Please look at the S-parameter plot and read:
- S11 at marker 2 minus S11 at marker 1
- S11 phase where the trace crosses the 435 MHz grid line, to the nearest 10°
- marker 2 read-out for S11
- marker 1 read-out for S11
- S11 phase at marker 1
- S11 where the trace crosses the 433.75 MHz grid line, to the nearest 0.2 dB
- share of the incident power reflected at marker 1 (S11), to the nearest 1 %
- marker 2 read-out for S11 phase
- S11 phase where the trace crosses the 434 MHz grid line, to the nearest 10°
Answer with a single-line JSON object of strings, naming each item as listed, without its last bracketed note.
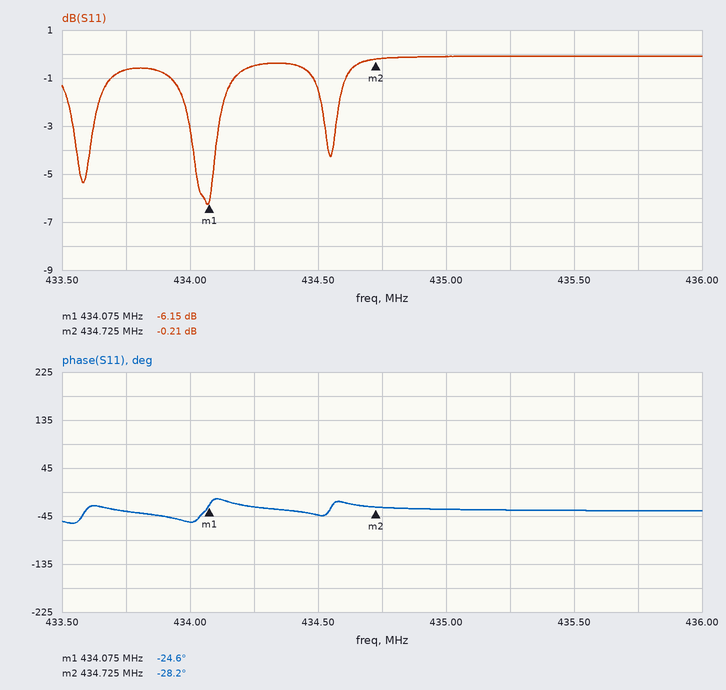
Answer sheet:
{"S11 at marker 2 minus S11 at marker 1": "5.94 dB", "S11 phase where the trace crosses the 435 MHz grid line, to the nearest 10°": "-30°", "marker 2 read-out for S11": "-0.21 dB", "marker 1 read-out for S11": "-6.15 dB", "S11 phase at marker 1": "-24.6°", "S11 where the trace crosses the 433.75 MHz grid line, to the nearest 0.2 dB": "-0.6 dB", "share of the incident power reflected at marker 1 (S11), to the nearest 1 %": "24 %", "marker 2 read-out for S11 phase": "-28.2°", "S11 phase where the trace crosses the 434 MHz grid line, to the nearest 10°": "-60°"}
